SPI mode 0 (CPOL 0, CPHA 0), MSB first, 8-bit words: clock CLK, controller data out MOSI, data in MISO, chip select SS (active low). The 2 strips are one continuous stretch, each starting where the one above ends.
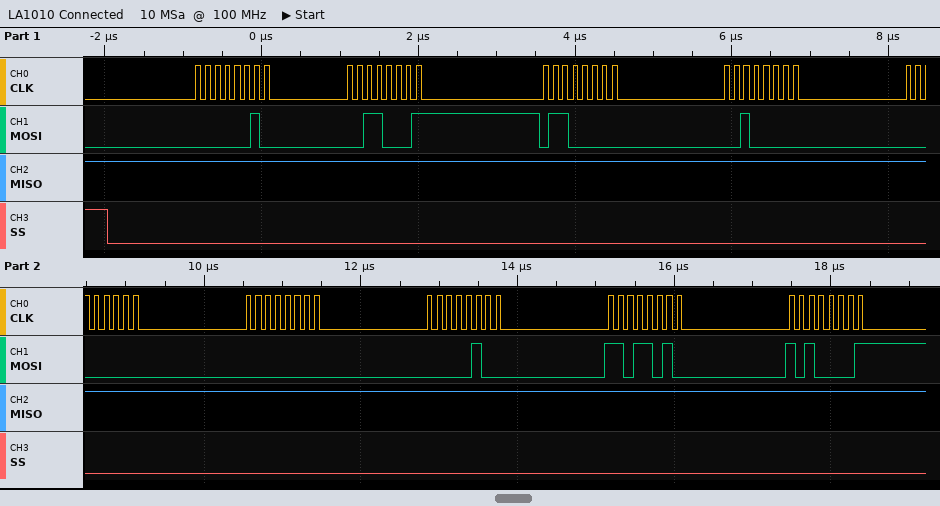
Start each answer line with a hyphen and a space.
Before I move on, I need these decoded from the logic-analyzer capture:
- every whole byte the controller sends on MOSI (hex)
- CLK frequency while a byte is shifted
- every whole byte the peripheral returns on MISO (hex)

- 02 31 60 20 00 00 04 DA A1
- 8 MHz
- FF FF FF FF FF FF FF FF FF
